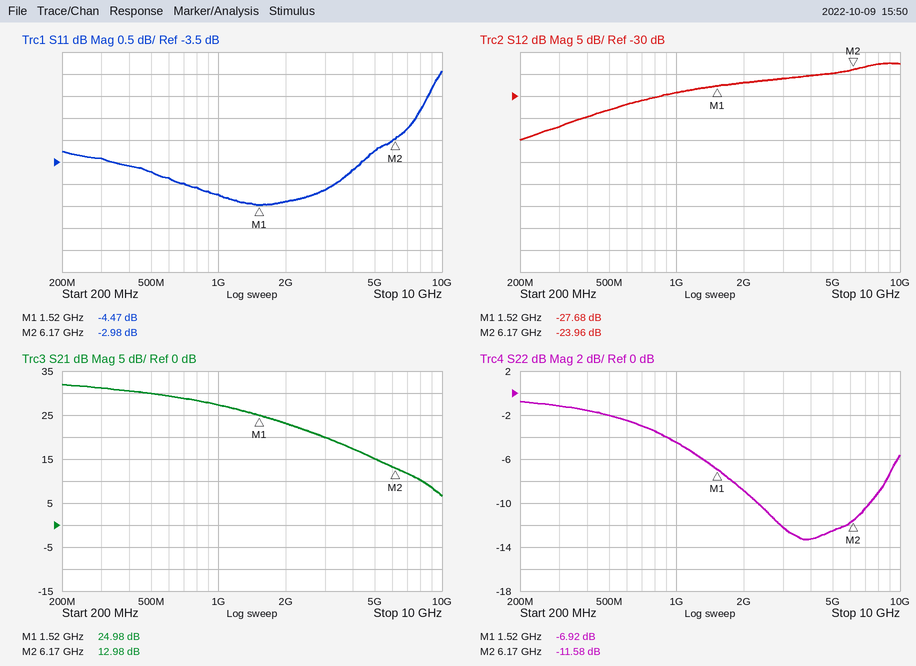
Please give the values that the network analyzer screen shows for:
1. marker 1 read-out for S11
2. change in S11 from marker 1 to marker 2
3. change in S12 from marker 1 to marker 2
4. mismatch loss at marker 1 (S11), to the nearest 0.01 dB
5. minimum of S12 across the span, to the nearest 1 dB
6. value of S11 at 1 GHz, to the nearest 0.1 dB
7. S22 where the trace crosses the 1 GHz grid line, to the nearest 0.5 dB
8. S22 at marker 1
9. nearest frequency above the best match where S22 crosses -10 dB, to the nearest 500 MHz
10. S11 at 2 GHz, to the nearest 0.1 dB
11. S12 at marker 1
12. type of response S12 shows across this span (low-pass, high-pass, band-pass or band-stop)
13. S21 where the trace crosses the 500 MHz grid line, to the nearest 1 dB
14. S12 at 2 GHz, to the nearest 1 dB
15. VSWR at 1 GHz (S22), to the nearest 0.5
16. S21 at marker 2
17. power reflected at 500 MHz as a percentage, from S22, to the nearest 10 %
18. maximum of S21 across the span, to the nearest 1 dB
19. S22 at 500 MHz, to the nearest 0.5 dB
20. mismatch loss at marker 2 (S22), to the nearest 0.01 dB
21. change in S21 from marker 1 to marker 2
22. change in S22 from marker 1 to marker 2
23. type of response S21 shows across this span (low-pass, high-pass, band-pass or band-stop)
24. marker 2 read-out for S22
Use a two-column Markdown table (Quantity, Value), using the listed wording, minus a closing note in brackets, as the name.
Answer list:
| Quantity | Value |
|---|---|
| marker 1 read-out for S11 | -4.47 dB |
| change in S11 from marker 1 to marker 2 | 1.49 dB |
| change in S12 from marker 1 to marker 2 | 3.72 dB |
| mismatch loss at marker 1 (S11), to the nearest 0.01 dB | 1.92 dB |
| minimum of S12 across the span, to the nearest 1 dB | -40 dB |
| value of S11 at 1 GHz, to the nearest 0.1 dB | -4.2 dB |
| S22 where the trace crosses the 1 GHz grid line, to the nearest 0.5 dB | -4.5 dB |
| S22 at marker 1 | -6.92 dB |
| nearest frequency above the best match where S22 crosses -10 dB, to the nearest 500 MHz | 7.5 GHz |
| S11 at 2 GHz, to the nearest 0.1 dB | -4.4 dB |
| S12 at marker 1 | -27.68 dB |
| type of response S12 shows across this span | high-pass |
| S21 where the trace crosses the 500 MHz grid line, to the nearest 1 dB | 30 dB |
| S12 at 2 GHz, to the nearest 1 dB | -27 dB |
| VSWR at 1 GHz (S22), to the nearest 0.5 | 4.0 |
| S21 at marker 2 | 12.98 dB |
| power reflected at 500 MHz as a percentage, from S22, to the nearest 10 % | 60 % |
| maximum of S21 across the span, to the nearest 1 dB | 32 dB |
| S22 at 500 MHz, to the nearest 0.5 dB | -2.0 dB |
| mismatch loss at marker 2 (S22), to the nearest 0.01 dB | 0.31 dB |
| change in S21 from marker 1 to marker 2 | -12.00 dB |
| change in S22 from marker 1 to marker 2 | -4.66 dB |
| type of response S21 shows across this span | low-pass |
| marker 2 read-out for S22 | -11.58 dB |
